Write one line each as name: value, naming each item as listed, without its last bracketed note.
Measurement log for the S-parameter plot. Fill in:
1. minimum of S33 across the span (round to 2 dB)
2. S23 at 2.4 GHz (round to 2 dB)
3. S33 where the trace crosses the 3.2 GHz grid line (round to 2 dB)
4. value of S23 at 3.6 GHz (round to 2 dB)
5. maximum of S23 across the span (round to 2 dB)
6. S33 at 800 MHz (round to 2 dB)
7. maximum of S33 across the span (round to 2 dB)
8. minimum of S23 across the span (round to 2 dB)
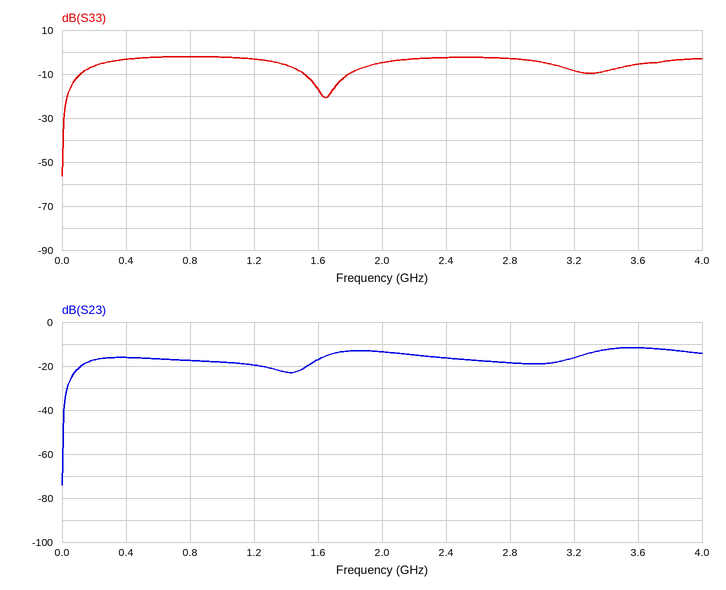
minimum of S33 across the span: -56 dB
S23 at 2.4 GHz: -16 dB
S33 where the trace crosses the 3.2 GHz grid line: -8 dB
value of S23 at 3.6 GHz: -12 dB
maximum of S23 across the span: -12 dB
S33 at 800 MHz: -2 dB
maximum of S33 across the span: -2 dB
minimum of S23 across the span: -74 dB
